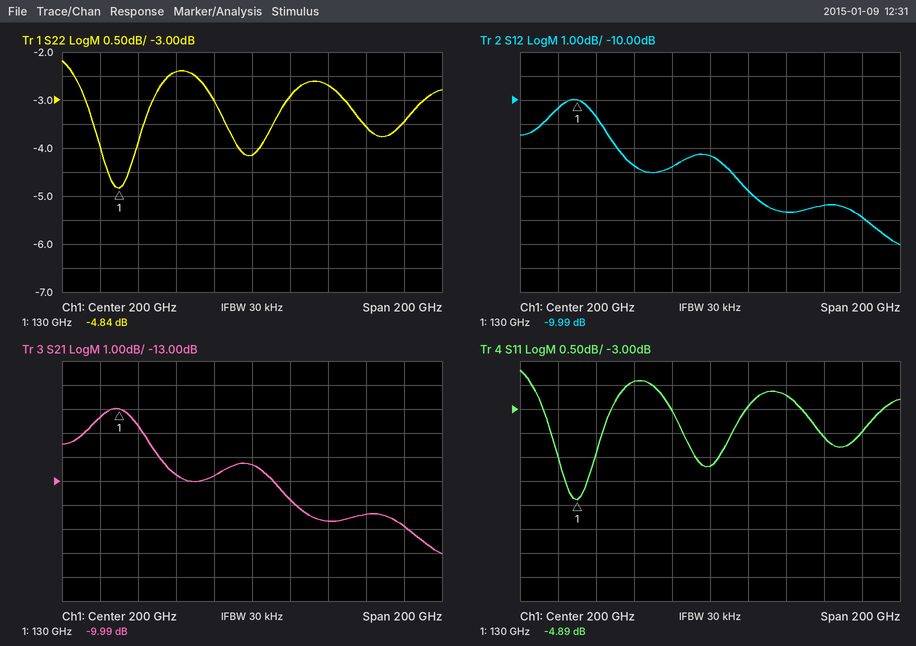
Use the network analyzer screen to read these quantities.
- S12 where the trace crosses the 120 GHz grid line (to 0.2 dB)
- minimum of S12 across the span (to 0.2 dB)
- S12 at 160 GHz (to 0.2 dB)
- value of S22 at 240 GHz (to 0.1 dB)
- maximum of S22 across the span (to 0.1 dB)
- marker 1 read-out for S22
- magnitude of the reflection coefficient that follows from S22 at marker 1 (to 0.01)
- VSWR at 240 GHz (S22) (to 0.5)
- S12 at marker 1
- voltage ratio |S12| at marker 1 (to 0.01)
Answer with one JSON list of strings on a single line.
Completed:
["-10.4 dB", "-16.0 dB", "-12.8 dB", "-2.7 dB", "-2.2 dB", "-4.84 dB", "0.57", "6.5", "-9.99 dB", "0.32"]
